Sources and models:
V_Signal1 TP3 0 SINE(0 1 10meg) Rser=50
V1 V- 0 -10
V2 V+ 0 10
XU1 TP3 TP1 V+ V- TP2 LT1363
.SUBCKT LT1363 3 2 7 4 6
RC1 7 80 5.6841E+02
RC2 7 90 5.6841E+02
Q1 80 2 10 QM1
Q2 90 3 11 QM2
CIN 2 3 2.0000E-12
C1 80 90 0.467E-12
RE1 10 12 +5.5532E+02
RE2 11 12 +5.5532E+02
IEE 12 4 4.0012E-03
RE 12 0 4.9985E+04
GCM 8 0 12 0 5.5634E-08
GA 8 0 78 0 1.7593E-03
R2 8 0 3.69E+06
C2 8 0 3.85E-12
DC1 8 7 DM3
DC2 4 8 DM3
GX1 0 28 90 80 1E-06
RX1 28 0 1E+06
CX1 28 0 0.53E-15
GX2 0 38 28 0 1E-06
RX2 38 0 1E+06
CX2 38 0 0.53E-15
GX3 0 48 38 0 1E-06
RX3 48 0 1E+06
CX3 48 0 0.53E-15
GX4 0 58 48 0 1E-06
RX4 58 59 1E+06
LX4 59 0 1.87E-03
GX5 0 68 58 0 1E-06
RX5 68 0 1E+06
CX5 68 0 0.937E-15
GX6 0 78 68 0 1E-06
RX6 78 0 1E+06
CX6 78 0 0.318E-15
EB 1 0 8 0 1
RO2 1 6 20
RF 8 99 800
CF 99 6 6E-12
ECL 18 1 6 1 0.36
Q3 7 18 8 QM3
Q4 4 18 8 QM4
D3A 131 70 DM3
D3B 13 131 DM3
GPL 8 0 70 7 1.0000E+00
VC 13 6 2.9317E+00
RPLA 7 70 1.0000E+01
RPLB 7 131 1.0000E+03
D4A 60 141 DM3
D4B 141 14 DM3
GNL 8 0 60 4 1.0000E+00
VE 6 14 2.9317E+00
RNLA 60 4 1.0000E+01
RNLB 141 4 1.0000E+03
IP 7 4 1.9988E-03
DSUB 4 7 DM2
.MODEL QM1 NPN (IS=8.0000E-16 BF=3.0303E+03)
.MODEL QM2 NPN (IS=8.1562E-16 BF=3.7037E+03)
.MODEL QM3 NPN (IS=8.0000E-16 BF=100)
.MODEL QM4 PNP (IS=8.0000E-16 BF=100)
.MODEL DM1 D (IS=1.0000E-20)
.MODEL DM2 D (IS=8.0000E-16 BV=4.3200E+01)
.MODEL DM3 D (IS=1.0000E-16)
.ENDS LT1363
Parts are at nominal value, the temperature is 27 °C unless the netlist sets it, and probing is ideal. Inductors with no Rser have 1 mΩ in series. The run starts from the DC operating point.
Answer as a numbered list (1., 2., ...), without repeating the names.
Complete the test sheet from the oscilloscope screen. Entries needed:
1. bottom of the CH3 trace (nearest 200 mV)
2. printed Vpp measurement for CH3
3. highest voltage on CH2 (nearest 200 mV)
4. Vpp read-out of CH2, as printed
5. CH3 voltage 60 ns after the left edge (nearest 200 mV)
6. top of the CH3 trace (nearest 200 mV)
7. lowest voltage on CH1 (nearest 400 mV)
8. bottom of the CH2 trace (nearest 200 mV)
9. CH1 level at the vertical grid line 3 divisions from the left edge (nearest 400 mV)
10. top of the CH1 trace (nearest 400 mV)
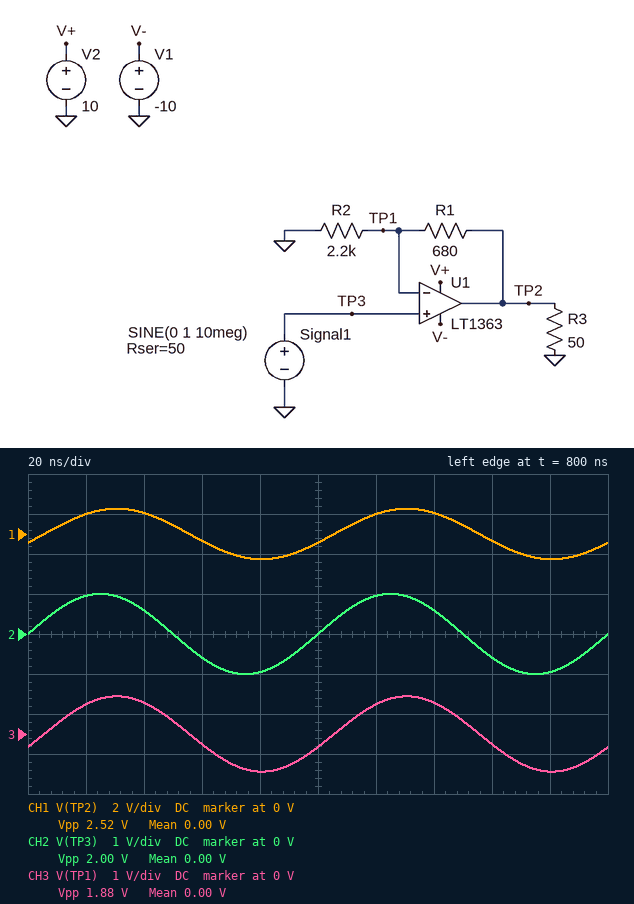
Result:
1. -1.0 V
2. 1.88 V
3. 1.0 V
4. 2.00 V
5. -200 mV
6. 1.0 V
7. -1.2 V
8. -1.0 V
9. -400 mV
10. 1.2 V
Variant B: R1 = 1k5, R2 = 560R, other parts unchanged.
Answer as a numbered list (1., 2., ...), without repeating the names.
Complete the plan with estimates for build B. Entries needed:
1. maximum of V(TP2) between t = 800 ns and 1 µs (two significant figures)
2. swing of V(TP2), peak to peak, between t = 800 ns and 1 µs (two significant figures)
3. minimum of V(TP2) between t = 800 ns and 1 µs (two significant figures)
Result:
1. 2.7 V
2. 5.3 V
3. -2.7 V
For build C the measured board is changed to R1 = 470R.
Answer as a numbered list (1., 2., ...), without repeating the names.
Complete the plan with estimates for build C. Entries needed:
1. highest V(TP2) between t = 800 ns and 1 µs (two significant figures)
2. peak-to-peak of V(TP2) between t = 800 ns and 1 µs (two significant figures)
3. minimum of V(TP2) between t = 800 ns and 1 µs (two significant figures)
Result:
1. 1.2 V
2. 2.3 V
3. -1.2 V
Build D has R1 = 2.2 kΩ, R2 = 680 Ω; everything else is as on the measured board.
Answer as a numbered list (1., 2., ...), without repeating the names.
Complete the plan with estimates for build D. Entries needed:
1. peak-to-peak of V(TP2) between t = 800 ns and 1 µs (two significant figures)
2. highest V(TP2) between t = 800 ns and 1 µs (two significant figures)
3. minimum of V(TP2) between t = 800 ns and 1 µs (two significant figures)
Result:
1. 5.7 V
2. 2.9 V
3. -2.9 V
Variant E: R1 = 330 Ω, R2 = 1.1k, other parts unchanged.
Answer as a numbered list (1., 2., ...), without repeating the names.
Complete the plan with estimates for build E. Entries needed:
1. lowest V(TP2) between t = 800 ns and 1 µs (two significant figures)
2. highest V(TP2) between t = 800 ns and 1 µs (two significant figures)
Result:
1. -1.2 V
2. 1.2 V
